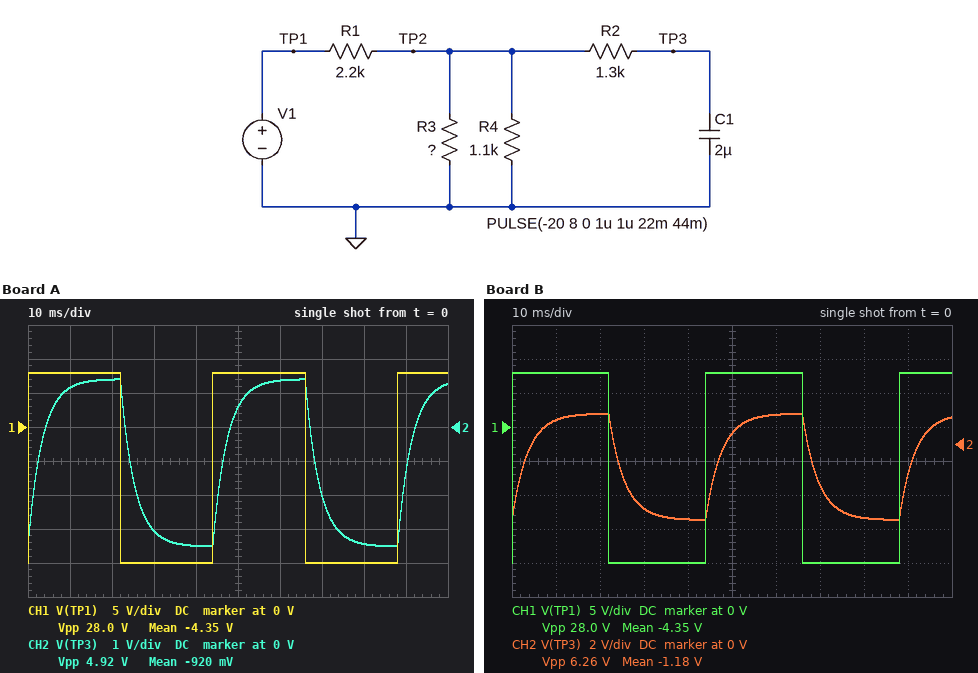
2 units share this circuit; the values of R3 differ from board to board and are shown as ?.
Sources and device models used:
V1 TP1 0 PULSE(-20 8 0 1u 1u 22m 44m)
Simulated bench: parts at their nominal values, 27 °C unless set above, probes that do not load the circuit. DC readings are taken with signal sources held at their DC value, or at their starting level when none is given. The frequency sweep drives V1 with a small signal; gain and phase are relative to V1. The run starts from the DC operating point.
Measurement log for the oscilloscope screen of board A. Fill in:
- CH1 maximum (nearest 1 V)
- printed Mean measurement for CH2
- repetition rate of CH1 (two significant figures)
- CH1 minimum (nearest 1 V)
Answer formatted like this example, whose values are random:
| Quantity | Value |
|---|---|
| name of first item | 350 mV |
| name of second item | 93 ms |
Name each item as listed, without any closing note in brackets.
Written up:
| Quantity | Value |
|---|---|
| CH1 maximum | 8 V |
| printed Mean measurement for CH2 | -920 mV |
| repetition rate of CH1 | 23 Hz |
| CH1 minimum | -20 V |
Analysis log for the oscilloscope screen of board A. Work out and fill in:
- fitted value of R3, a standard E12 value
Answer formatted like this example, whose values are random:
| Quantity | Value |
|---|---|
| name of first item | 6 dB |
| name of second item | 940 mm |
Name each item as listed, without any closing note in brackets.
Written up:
| Quantity | Value |
|---|---|
| fitted value of R3, a standard E12 value | 820 Ω |
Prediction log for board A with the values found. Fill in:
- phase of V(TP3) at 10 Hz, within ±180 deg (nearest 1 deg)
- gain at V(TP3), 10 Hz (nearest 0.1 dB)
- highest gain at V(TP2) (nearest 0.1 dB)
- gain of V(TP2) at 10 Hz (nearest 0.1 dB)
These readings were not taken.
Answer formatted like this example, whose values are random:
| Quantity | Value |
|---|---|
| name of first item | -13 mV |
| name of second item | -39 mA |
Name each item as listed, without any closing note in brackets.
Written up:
| Quantity | Value |
|---|---|
| phase of V(TP3) at 10 Hz, within ±180 deg | -12 deg |
| gain at V(TP3), 10 Hz | -15.3 dB |
| highest gain at V(TP2) | -15.1 dB |
| gain of V(TP2) at 10 Hz | -15.2 dB |
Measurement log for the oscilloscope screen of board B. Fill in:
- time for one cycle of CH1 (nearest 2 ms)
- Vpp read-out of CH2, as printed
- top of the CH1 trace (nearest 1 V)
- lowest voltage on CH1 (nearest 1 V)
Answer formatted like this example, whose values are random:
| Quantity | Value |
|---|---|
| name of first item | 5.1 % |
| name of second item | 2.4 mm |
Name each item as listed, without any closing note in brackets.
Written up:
| Quantity | Value |
|---|---|
| time for one cycle of CH1 | 44 ms |
| Vpp read-out of CH2, as printed | 6.26 V |
| top of the CH1 trace | 8 V |
| lowest voltage on CH1 | -20 V |
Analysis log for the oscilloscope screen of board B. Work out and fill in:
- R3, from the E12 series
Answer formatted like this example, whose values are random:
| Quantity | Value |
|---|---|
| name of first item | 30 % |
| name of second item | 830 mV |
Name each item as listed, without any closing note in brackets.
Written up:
| Quantity | Value |
|---|---|
| R3, from the E12 series | 1.5 kΩ |
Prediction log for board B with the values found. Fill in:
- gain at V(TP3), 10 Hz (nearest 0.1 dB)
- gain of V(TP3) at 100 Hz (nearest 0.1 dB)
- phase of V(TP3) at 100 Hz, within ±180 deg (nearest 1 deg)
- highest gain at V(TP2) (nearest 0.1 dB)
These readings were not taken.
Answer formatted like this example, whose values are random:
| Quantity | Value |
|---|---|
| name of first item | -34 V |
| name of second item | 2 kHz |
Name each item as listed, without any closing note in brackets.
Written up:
| Quantity | Value |
|---|---|
| gain at V(TP3), 10 Hz | -13.2 dB |
| gain of V(TP3) at 100 Hz | -20.8 dB |
| phase of V(TP3) at 100 Hz, within ±180 deg | -66 deg |
| highest gain at V(TP2) | -13.0 dB |
